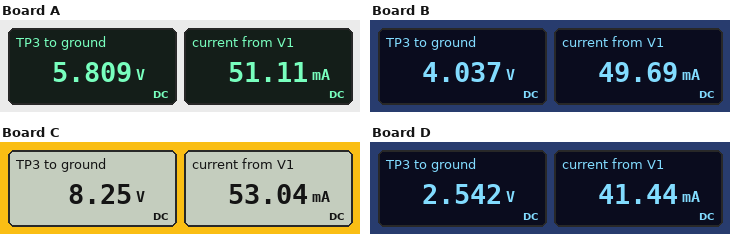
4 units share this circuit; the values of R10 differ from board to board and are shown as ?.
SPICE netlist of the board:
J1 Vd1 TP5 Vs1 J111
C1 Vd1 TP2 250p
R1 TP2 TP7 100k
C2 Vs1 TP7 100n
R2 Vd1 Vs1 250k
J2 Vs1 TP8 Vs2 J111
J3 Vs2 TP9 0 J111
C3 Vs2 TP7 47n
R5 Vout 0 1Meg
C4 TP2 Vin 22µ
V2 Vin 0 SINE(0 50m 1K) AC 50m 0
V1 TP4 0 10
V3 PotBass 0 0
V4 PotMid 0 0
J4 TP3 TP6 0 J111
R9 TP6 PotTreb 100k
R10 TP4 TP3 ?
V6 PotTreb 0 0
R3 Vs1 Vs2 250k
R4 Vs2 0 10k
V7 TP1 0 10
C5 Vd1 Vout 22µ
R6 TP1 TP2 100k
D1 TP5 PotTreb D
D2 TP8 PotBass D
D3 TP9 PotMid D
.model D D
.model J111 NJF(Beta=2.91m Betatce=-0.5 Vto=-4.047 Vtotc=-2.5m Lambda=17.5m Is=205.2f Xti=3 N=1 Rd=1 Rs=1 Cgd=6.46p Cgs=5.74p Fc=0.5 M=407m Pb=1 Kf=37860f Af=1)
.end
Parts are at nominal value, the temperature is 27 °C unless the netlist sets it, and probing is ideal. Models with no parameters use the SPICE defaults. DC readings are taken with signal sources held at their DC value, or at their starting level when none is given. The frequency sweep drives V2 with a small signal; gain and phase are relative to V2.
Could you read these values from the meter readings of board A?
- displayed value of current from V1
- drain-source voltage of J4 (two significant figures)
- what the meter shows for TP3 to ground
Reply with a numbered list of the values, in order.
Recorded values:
1. 51.11 mA
2. 5.8 V
3. 5.809 V
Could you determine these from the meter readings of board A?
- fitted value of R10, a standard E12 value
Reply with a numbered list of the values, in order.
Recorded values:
1. 82 Ω
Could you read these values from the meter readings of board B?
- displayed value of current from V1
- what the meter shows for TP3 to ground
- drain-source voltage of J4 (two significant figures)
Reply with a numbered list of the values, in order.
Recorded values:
1. 49.69 mA
2. 4.037 V
3. 4.0 V
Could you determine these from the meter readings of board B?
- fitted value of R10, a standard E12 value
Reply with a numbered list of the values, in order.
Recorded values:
1. 120 Ω
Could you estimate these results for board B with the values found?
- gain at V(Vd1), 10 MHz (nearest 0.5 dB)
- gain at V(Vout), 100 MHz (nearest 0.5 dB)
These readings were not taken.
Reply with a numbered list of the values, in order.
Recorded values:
1. -2.0 dB
2. 0 dB
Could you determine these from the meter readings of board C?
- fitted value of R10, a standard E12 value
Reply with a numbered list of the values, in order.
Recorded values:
1. 33 Ω
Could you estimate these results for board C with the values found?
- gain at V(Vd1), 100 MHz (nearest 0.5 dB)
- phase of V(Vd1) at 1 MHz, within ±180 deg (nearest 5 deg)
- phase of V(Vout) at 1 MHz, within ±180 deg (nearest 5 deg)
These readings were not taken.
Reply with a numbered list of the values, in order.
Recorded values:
1. 0 dB
2. 80 deg
3. 80 deg
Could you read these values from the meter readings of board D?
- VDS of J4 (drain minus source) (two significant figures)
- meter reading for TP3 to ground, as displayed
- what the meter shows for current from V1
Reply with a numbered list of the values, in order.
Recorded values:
1. 2.5 V
2. 2.542 V
3. 41.44 mA
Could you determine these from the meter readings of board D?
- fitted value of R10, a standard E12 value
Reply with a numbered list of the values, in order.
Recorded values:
1. 180 Ω
